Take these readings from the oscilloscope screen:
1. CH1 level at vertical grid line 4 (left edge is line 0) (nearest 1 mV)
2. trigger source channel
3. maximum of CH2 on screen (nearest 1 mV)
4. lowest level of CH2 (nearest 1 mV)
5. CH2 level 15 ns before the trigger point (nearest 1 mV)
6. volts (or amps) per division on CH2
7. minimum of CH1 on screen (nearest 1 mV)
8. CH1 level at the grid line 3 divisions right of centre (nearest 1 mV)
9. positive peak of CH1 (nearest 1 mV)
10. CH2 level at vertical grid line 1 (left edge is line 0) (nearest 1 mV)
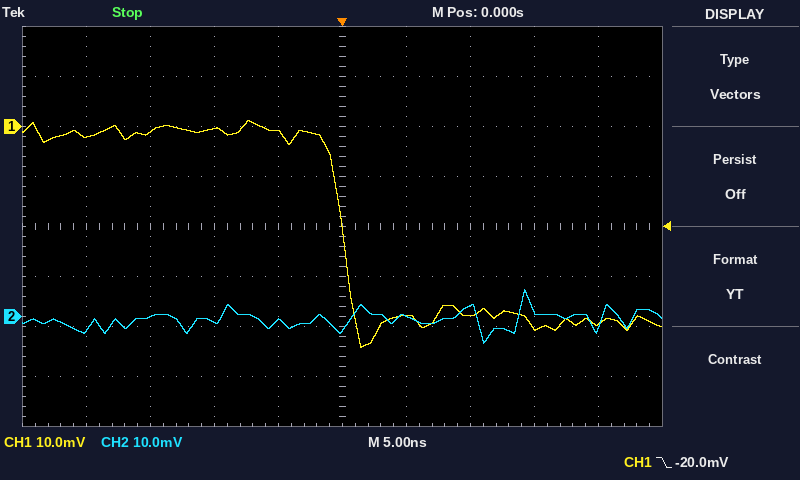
-1 mV
CH1
5 mV
-5 mV
0 mV
10 mV
-44 mV
-40 mV
1 mV
-3 mV
